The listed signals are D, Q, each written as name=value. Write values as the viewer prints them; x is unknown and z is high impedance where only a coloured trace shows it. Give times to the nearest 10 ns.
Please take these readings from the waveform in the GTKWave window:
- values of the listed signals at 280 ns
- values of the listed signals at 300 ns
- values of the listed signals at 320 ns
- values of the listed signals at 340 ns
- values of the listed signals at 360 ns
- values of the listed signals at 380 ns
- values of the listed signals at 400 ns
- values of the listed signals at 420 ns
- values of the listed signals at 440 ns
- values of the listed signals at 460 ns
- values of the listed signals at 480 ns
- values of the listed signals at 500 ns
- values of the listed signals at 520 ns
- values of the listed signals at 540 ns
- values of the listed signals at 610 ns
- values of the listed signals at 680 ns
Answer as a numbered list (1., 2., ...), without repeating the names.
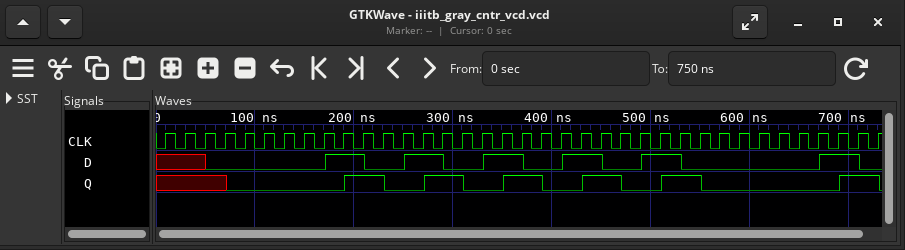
1. D=1, Q=1
2. D=0, Q=1
3. D=0, Q=0
4. D=1, Q=0
5. D=1, Q=1
6. D=0, Q=1
7. D=0, Q=0
8. D=1, Q=0
9. D=1, Q=1
10. D=0, Q=1
11. D=0, Q=0
12. D=1, Q=0
13. D=1, Q=1
14. D=0, Q=1
15. D=0, Q=0
16. D=1, Q=0
